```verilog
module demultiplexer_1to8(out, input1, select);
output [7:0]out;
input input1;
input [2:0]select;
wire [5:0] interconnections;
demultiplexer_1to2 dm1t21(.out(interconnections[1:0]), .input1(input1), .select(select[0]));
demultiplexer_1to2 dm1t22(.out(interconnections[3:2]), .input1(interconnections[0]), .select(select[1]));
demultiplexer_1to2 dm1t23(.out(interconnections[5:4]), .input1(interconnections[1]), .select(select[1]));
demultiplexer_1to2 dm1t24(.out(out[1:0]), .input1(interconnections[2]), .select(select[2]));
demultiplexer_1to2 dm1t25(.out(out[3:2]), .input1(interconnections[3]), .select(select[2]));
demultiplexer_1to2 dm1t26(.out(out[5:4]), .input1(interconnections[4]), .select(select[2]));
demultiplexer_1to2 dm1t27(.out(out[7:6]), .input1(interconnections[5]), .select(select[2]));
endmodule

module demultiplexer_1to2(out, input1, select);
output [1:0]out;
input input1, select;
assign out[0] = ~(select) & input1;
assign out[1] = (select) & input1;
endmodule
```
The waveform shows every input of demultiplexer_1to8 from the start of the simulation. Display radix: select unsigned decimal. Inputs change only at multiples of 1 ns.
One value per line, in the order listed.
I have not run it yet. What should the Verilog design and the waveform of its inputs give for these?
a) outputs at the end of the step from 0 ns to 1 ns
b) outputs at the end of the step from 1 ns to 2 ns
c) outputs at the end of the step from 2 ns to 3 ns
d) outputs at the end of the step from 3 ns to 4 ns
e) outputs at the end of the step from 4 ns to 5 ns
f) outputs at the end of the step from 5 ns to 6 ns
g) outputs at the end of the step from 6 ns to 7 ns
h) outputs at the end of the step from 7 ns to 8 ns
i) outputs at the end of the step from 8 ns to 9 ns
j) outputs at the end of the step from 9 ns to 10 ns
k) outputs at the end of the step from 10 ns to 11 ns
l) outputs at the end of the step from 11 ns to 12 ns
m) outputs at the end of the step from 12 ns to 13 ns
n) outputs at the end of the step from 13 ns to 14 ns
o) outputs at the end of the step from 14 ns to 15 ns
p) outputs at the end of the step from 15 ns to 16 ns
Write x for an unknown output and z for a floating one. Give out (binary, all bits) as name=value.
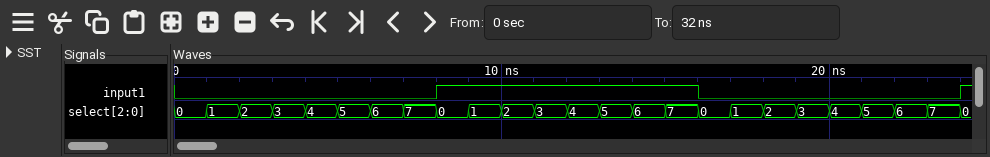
out=00000000
out=00000000
out=00000000
out=00000000
out=00000000
out=00000000
out=00000000
out=00000000
out=00000001
out=00010000
out=00000100
out=01000000
out=00000010
out=00100000
out=00001000
out=10000000
